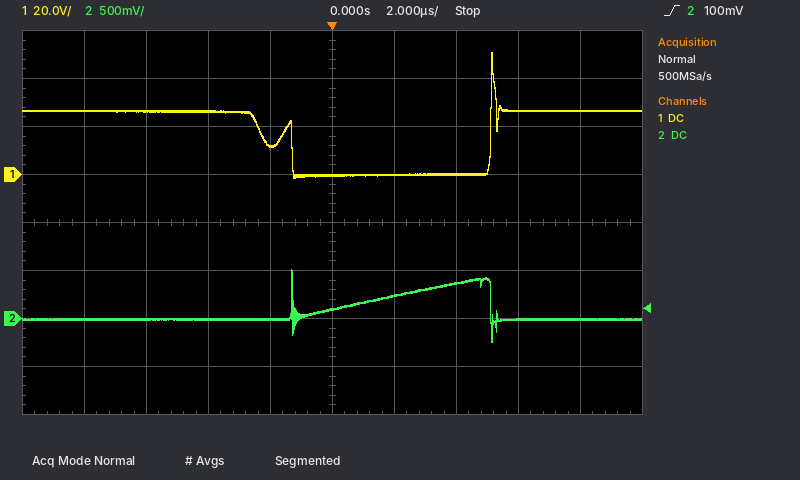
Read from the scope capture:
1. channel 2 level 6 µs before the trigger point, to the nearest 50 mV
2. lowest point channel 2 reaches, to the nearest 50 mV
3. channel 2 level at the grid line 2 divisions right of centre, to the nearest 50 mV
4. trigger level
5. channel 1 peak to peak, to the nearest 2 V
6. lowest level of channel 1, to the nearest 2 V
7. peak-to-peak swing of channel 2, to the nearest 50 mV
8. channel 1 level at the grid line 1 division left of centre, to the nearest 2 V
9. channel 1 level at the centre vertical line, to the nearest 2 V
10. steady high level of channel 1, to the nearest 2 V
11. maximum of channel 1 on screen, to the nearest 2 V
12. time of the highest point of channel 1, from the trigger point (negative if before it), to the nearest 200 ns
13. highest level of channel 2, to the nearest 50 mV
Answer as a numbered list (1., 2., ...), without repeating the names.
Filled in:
1. 0 mV
2. -250 mV
3. 350 mV
4. 100 mV
5. 52 V
6. -2 V
7. 750 mV
8. 12 V
9. 0 V
10. 26 V
11. 50 V
12. +5.2 µs
13. 500 mV
